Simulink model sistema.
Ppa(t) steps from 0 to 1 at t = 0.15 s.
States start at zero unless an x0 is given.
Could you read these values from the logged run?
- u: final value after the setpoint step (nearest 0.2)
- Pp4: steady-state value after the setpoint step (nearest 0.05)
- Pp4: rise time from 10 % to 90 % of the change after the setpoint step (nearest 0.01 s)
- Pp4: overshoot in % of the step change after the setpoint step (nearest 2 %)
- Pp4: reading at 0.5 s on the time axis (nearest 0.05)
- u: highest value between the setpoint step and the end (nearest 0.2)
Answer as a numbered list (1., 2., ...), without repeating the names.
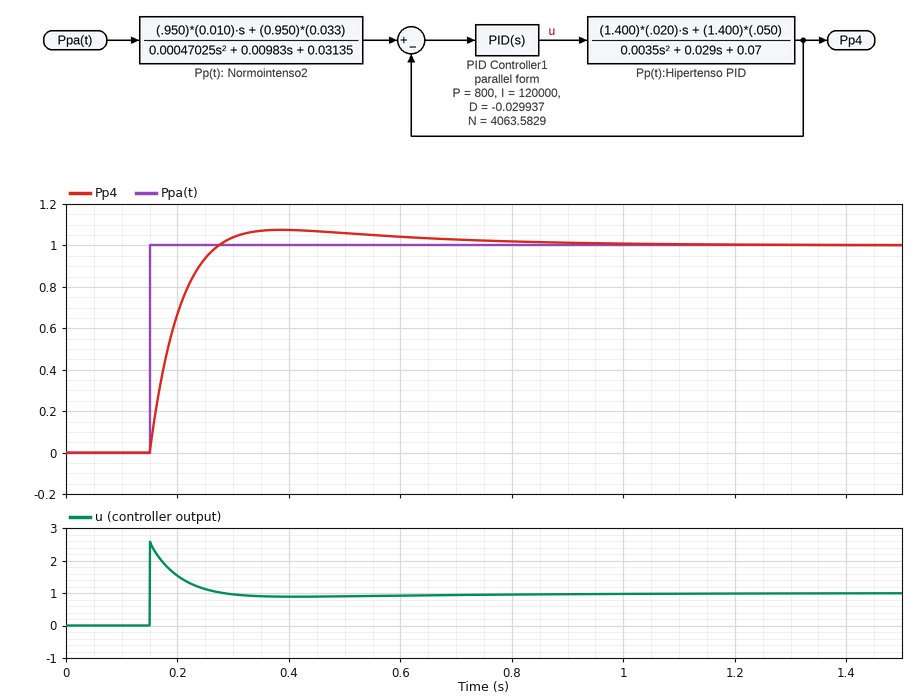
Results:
1. 1.0
2. 1.00
3. 0.08 s
4. 8 %
5. 1.05
6. 2.6
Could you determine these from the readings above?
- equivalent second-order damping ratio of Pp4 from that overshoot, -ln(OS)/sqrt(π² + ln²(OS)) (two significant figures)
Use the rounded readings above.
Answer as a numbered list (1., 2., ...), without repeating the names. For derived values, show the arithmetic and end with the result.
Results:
1. ln(0.08) = -2.526; 2.526 / sqrt(9.870 + 6.379) = 0.63
